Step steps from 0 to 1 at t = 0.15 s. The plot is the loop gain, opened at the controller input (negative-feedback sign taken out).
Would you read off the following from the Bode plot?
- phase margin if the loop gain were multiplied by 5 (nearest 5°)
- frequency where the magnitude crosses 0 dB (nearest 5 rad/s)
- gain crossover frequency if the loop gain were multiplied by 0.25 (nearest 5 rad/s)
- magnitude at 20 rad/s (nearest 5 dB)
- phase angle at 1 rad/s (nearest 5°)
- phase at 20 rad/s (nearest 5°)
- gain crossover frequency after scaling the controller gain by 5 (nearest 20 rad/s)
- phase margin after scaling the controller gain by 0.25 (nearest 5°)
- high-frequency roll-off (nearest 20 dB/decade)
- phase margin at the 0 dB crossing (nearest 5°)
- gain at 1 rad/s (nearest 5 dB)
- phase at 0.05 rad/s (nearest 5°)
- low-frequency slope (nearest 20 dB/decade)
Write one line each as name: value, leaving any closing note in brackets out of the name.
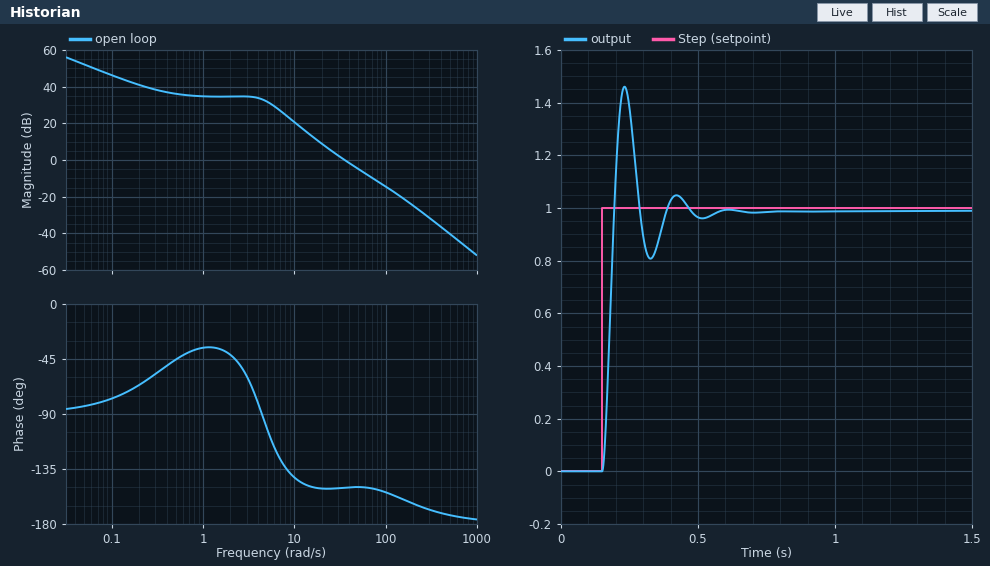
phase margin if the loop gain were multiplied by 5: 25°
frequency where the magnitude crosses 0 dB: 35 rad/s
gain crossover frequency if the loop gain were multiplied by 0.25: 15 rad/s
magnitude at 20 rad/s: 10 dB
phase angle at 1 rad/s: -35°
phase at 20 rad/s: -150°
gain crossover frequency after scaling the controller gain by 5: 100 rad/s
phase margin after scaling the controller gain by 0.25: 30°
high-frequency roll-off: -40 dB/decade
phase margin at the 0 dB crossing: 30°
gain at 1 rad/s: 35 dB
phase at 0.05 rad/s: -85°
low-frequency slope: -20 dB/decade
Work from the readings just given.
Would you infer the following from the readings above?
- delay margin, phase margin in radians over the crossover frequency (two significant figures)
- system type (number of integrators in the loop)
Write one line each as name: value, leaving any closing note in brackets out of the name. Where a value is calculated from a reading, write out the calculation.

delay margin, phase margin in radians over the crossover frequency: 30 × π / 180 / 35 = 0.015 s
system type: 1
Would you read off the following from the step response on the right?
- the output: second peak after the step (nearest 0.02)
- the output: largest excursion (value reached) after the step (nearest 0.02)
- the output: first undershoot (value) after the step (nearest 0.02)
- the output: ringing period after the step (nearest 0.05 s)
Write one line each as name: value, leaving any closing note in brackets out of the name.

the output: second peak after the step: 1.04
the output: largest excursion (value reached) after the step: 1.46
the output: first undershoot (value) after the step: 0.80
the output: ringing period after the step: 0.20 s
